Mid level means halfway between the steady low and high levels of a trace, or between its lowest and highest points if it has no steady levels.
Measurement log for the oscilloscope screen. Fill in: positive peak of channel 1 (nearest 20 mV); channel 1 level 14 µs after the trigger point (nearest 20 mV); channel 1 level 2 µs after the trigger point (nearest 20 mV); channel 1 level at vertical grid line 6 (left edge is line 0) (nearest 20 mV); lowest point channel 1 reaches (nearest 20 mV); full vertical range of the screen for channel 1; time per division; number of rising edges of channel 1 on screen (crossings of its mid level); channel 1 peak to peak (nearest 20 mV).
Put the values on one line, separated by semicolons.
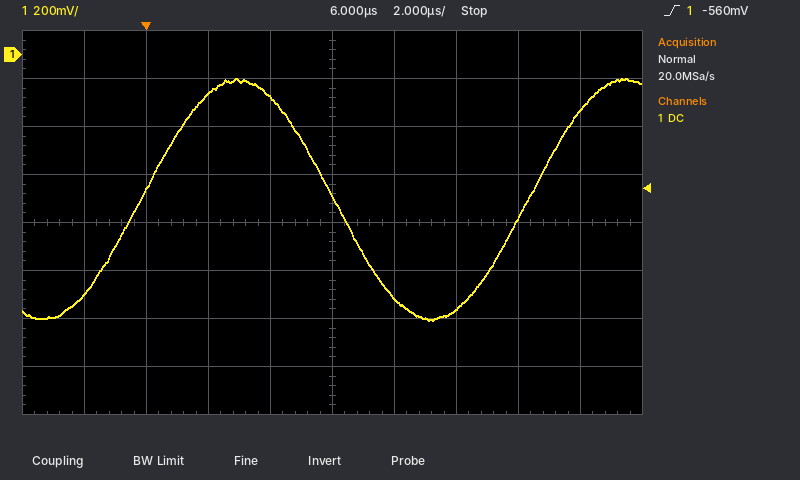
-100 mV; -240 mV; -160 mV; -1.02 V; -1.10 V; 1.6 V; 2 µs; 2; 1.00 V
